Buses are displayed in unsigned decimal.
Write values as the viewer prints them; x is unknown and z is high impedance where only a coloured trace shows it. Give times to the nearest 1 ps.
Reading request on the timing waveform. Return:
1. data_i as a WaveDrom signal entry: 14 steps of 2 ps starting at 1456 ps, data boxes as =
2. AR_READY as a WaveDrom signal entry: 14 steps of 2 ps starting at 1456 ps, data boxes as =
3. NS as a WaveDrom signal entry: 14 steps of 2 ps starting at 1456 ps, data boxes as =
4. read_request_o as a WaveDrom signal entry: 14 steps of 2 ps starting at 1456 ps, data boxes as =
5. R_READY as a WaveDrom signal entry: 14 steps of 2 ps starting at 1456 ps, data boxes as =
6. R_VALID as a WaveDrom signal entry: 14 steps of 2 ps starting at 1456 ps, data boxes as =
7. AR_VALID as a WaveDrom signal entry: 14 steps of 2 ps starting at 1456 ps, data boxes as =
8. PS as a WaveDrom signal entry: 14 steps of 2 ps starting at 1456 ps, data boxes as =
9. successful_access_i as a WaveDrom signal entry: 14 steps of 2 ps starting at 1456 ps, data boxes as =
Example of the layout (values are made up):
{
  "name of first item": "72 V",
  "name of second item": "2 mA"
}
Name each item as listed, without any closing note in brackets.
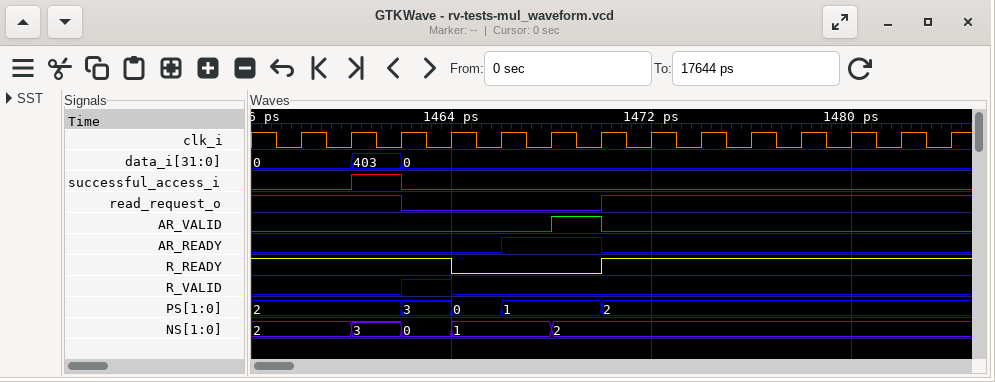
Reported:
{
  "data_i as a WaveDrom signal entry: 14 steps of 2 ps starting at 1456 ps, data boxes as =": "{name: 'data_i', wave: '=.==..........', data: '0 403 0'}",
  "AR_READY as a WaveDrom signal entry: 14 steps of 2 ps starting at 1456 ps, data boxes as =": "{name: 'AR_READY', wave: '0....1.0......'}",
  "NS as a WaveDrom signal entry: 14 steps of 2 ps starting at 1456 ps, data boxes as =": "{name: 'NS', wave: '=.===.=.......', data: '2 3 0 1 2'}",
  "read_request_o as a WaveDrom signal entry: 14 steps of 2 ps starting at 1456 ps, data boxes as =": "{name: 'read_request_o', wave: '1..0...1......'}",
  "R_READY as a WaveDrom signal entry: 14 steps of 2 ps starting at 1456 ps, data boxes as =": "{name: 'R_READY', wave: '1...0..1......'}",
  "R_VALID as a WaveDrom signal entry: 14 steps of 2 ps starting at 1456 ps, data boxes as =": "{name: 'R_VALID', wave: '0..10.........'}",
  "AR_VALID as a WaveDrom signal entry: 14 steps of 2 ps starting at 1456 ps, data boxes as =": "{name: 'AR_VALID', wave: '0.....10......'}",
  "PS as a WaveDrom signal entry: 14 steps of 2 ps starting at 1456 ps, data boxes as =": "{name: 'PS', wave: '=..===.=......', data: '2 3 0 1 2'}",
  "successful_access_i as a WaveDrom signal entry: 14 steps of 2 ps starting at 1456 ps, data boxes as =": "{name: 'successful_access_i', wave: '0.10..........'}"
}
